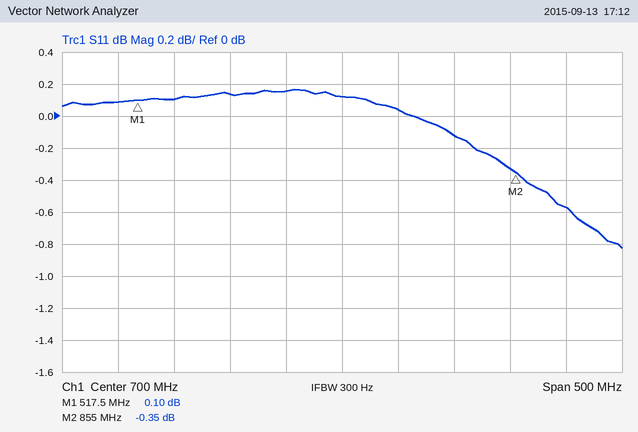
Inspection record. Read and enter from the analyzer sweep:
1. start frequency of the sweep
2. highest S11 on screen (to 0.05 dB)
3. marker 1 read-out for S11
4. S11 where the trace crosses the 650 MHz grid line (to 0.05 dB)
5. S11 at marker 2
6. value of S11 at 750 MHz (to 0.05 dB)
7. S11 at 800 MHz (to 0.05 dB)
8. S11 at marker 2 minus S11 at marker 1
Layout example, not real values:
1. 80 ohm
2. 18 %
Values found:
1. 450 MHz
2. 0.15 dB
3. 0.10 dB
4. 0.15 dB
5. -0.35 dB
6. 0.05 dB
7. -0.10 dB
8. -0.45 dB
